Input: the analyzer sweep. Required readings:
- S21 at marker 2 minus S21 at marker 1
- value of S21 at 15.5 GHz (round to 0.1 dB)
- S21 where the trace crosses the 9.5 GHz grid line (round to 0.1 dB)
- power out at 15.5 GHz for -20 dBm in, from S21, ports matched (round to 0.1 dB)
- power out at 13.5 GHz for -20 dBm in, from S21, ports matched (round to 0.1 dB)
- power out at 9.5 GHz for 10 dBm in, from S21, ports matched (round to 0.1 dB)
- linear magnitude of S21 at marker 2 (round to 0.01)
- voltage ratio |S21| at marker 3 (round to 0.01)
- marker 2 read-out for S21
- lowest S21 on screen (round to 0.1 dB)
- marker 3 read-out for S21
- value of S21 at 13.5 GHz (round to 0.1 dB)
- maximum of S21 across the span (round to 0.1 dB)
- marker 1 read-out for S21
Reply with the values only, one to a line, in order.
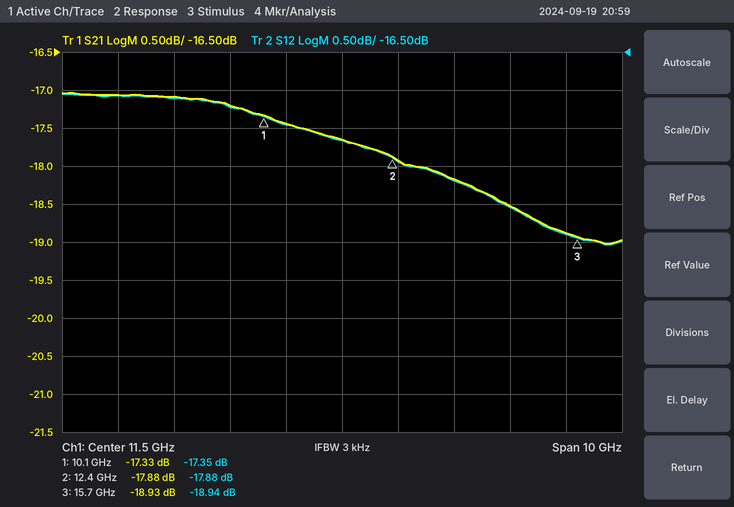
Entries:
-0.55 dB
-18.9 dB
-17.2 dB
-38.9 dBm
-38.2 dBm
-7.2 dBm
0.13
0.11
-17.88 dB
-19.0 dB
-18.93 dB
-18.2 dB
-17.0 dB
-17.33 dB
